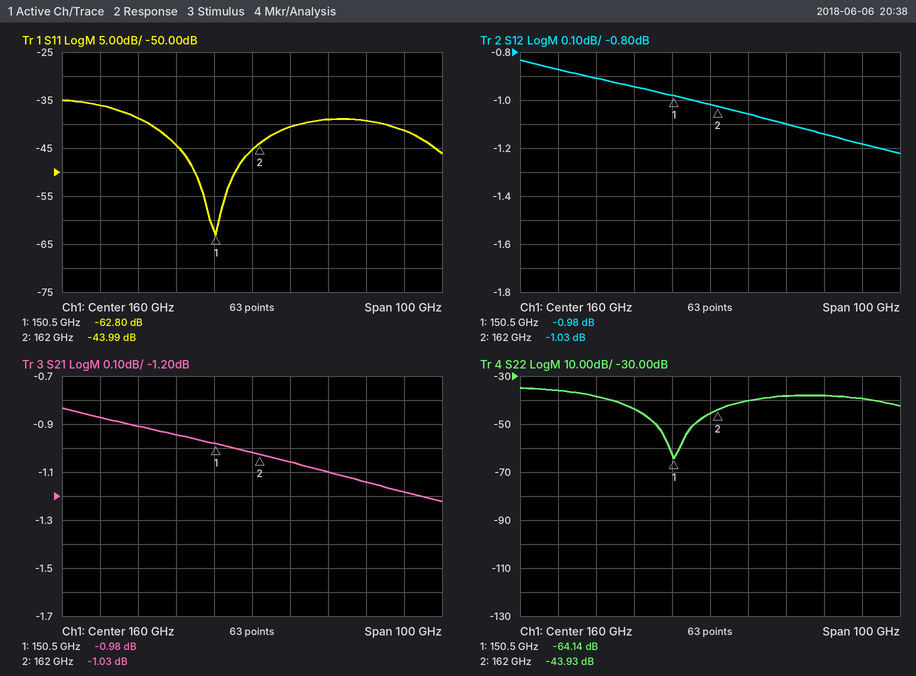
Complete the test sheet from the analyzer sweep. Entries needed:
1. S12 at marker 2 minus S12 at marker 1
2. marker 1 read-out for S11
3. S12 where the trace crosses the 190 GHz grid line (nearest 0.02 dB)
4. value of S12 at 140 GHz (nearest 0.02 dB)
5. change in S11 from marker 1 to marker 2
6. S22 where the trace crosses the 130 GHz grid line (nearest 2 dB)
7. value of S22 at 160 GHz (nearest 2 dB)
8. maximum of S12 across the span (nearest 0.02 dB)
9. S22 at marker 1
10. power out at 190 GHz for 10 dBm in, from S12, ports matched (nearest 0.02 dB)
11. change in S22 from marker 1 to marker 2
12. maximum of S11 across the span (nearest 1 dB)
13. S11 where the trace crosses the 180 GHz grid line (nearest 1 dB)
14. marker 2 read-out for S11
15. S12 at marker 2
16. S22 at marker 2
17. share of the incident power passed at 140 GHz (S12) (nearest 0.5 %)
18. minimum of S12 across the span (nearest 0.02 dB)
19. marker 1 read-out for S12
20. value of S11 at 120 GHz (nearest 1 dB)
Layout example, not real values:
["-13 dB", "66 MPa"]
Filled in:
["-0.05 dB", "-62.80 dB", "-1.14 dB", "-0.94 dB", "18.81 dB", "-38 dB", "-46 dB", "-0.84 dB", "-64.14 dB", "8.86 dBm", "20.21 dB", "-35 dB", "-39 dB", "-43.99 dB", "-1.03 dB", "-43.93 dB", "80.5 %", "-1.22 dB", "-0.98 dB", "-36 dB"]
